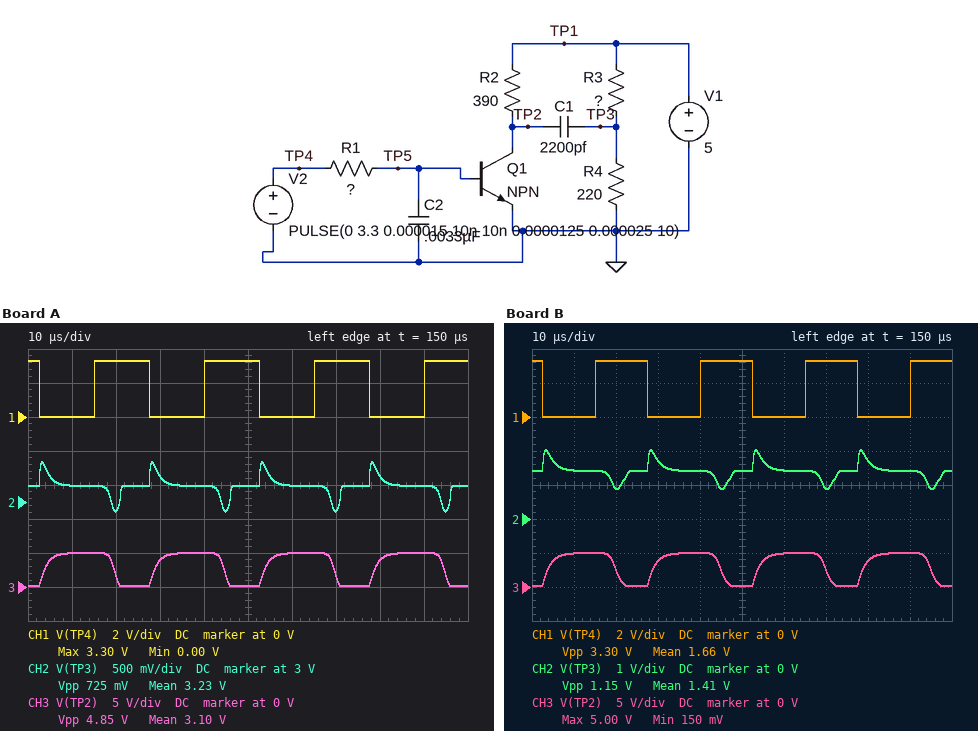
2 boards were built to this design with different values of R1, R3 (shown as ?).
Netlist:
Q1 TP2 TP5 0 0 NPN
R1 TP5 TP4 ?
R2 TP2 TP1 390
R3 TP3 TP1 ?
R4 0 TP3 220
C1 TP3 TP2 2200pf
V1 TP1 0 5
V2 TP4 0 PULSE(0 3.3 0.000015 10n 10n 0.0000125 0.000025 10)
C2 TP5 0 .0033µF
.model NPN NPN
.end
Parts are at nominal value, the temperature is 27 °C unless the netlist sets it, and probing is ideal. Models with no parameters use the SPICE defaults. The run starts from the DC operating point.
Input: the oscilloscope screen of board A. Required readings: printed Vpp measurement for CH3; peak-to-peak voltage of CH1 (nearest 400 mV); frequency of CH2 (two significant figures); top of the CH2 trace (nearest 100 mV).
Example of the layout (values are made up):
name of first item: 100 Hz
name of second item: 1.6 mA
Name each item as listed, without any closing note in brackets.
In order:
printed Vpp measurement for CH3: 4.85 V
peak-to-peak voltage of CH1: 3.2 V
frequency of CH2: 40 kHz
top of the CH2 trace: 3.6 V
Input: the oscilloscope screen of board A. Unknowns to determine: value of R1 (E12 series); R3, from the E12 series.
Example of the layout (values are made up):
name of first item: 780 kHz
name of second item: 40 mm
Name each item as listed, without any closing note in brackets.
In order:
value of R1: 15 kΩ
R3, from the E12 series: 120 Ω
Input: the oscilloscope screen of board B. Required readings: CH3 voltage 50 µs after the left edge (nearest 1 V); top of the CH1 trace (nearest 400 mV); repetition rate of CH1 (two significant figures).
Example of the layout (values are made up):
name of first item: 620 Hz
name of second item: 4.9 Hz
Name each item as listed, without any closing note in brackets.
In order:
CH3 voltage 50 µs after the left edge: 0 V
top of the CH1 trace: 3.2 V
repetition rate of CH1: 40 kHz
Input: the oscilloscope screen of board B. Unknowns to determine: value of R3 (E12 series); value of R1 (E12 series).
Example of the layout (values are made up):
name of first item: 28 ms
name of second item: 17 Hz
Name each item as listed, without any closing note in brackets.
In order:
value of R3: 560 Ω
value of R1: 18 kΩ
